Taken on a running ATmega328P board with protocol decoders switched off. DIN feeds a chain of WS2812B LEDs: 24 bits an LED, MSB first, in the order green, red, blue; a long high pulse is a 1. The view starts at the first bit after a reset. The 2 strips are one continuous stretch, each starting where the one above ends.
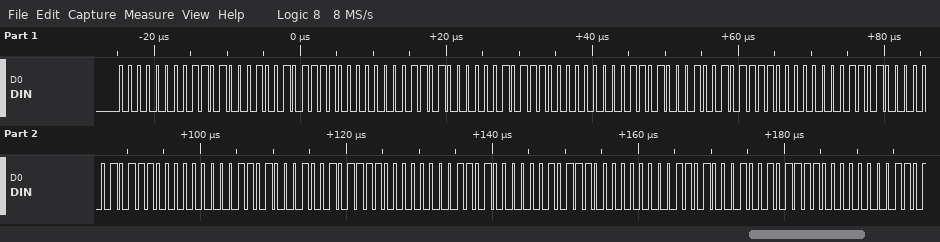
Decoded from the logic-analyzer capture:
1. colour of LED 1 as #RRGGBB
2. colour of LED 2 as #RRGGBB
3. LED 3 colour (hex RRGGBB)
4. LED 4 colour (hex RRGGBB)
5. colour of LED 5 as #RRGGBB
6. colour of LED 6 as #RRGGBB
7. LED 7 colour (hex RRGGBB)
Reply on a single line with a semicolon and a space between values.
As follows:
#D1002F; #D0002E; #D1002F; #D0002E; #D1002F; #D0002E; #D1002F
